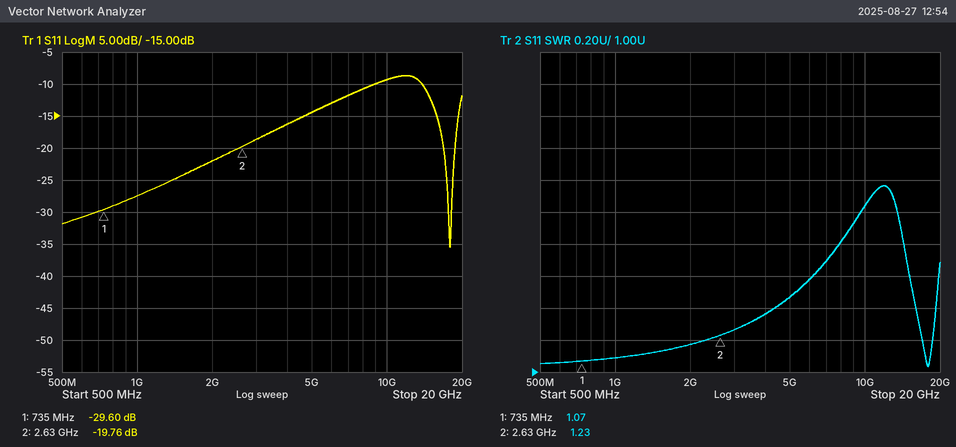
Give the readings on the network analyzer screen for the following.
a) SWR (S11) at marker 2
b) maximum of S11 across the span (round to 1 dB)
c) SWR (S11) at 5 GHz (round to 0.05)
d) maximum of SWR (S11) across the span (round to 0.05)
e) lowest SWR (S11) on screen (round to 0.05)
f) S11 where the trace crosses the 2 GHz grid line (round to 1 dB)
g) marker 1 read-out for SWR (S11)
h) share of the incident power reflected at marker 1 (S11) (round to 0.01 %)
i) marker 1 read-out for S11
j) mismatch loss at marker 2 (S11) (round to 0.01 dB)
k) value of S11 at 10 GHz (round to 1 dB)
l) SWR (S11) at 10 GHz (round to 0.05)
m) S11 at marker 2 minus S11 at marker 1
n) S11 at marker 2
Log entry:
1.23
-9 dB
1.45
2.15
1.05
-22 dB
1.07
0.11 %
-29.60 dB
0.05 dB
-9 dB
2.05
9.84 dB
-19.76 dB
